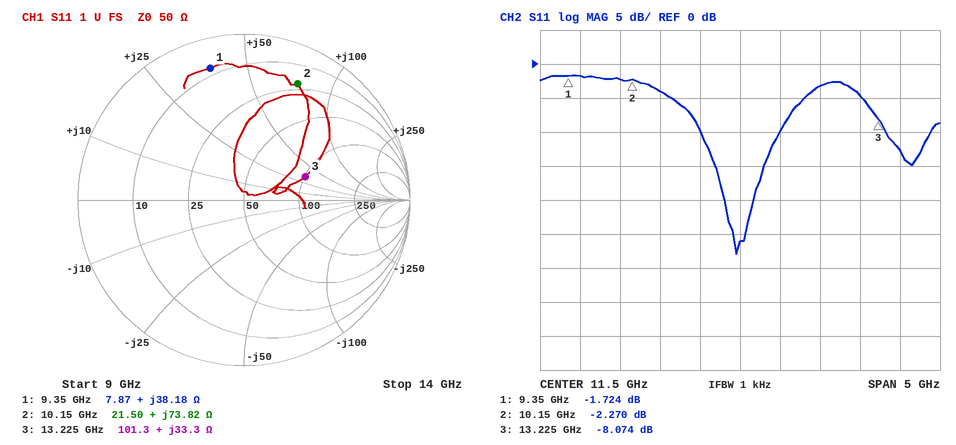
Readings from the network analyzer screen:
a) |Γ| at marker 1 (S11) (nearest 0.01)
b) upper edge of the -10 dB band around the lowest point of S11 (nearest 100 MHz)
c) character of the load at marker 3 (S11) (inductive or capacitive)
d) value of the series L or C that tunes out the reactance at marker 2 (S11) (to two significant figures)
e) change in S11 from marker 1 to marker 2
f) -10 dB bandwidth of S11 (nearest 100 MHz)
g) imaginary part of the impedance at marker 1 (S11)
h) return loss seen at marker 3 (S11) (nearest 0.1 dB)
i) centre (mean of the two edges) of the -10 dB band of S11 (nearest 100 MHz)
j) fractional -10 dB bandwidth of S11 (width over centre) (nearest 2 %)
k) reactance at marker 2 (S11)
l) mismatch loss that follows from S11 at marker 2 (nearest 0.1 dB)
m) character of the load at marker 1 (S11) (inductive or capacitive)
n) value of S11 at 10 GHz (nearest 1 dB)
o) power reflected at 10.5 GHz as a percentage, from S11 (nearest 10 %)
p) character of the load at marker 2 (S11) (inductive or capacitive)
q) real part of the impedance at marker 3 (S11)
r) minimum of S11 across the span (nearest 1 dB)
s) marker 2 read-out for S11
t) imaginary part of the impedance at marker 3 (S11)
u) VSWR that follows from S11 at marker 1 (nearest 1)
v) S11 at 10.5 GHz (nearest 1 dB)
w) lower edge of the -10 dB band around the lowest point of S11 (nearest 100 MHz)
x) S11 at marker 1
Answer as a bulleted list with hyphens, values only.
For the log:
- 0.82
- 12.0 GHz
- inductive
- 210 fF
- -0.546 dB
- 1.0 GHz
- +38.18 Ω
- 8.1 dB
- 11.5 GHz
- 8 %
- +73.82 Ω
- 3.9 dB
- inductive
- -2 dB
- 40 %
- inductive
- 101.3 Ω
- -28 dB
- -2.270 dB
- +33.3 Ω
- 10
- -4 dB
- 11.0 GHz
- -1.724 dB
